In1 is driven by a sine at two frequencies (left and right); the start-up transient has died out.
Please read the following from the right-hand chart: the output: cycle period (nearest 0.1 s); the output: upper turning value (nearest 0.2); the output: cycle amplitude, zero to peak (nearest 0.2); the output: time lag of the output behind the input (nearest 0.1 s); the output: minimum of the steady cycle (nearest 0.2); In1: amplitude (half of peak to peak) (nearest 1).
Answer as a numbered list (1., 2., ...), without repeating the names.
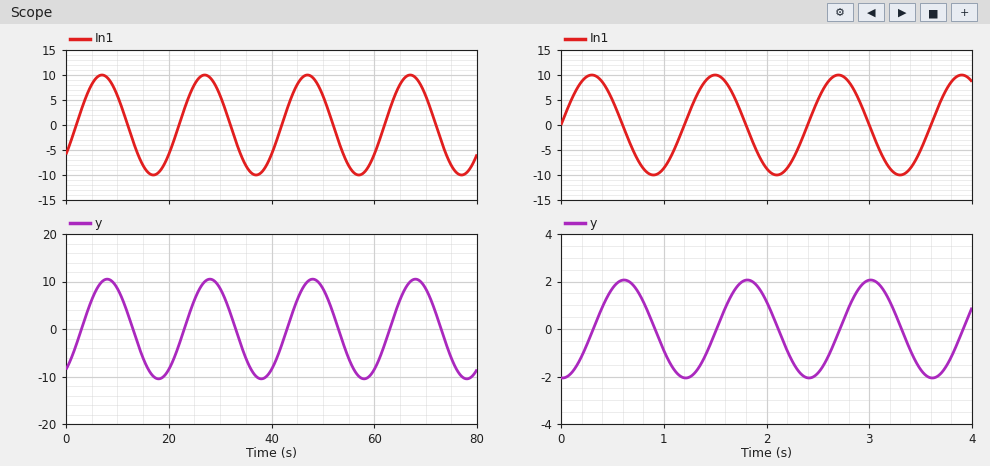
1. 1.2 s
2. 2.0
3. 2.0
4. 0.3 s
5. -2.0
6. 10
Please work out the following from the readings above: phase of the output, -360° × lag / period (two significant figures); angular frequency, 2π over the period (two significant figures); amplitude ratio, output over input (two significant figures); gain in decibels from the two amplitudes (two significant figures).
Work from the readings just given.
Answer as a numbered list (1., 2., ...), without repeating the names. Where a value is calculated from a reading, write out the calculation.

1. -360 × 0.3 / 1.2 = -90°
2. 2π / 1.2 = 5.2 rad/s
3. 2 / 10 = 0.20
4. 20 log10(2 / 10) = -14 dB
